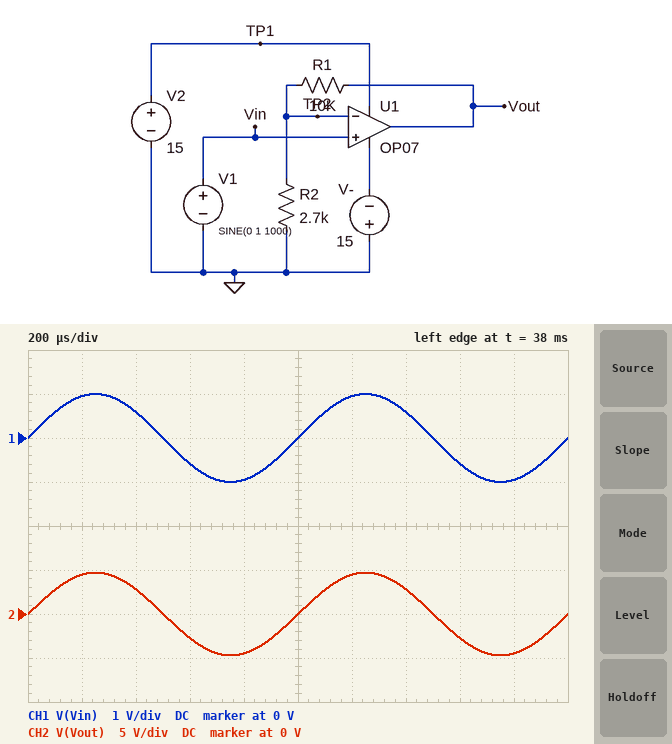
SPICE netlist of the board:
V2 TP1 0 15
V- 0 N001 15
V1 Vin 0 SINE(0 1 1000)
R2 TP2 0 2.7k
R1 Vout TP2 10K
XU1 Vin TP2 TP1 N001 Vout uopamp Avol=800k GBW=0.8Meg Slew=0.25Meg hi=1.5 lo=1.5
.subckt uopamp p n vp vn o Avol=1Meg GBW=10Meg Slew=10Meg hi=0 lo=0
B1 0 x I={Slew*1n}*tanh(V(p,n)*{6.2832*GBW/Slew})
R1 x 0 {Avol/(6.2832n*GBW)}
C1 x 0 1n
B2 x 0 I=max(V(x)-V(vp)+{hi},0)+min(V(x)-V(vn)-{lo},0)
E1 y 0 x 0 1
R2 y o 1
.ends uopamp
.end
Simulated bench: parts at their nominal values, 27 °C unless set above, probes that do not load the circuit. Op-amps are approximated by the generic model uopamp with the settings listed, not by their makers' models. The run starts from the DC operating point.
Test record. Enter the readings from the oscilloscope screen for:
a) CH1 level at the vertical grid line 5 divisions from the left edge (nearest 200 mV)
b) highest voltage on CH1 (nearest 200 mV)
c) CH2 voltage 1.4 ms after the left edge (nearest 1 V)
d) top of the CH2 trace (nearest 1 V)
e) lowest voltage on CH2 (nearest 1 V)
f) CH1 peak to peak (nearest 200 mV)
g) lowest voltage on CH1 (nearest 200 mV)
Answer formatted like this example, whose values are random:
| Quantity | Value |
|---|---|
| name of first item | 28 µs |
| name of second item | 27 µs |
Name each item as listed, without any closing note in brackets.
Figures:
| Quantity | Value |
|---|---|
| CH1 level at the vertical grid line 5 divisions from the left edge | 0 V |
| highest voltage on CH1 | 1.0 V |
| CH2 voltage 1.4 ms after the left edge | 3 V |
| top of the CH2 trace | 5 V |
| lowest voltage on CH2 | -5 V |
| CH1 peak to peak | 2.0 V |
| lowest voltage on CH1 | -1.0 V |
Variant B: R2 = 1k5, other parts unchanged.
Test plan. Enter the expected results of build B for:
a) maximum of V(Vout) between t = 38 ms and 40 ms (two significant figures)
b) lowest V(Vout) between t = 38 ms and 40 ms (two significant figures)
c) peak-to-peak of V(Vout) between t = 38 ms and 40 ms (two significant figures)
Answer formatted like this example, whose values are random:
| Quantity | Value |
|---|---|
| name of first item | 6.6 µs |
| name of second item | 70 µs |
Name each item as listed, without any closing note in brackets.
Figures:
| Quantity | Value |
|---|---|
| maximum of V(Vout) between t = 38 ms and 40 ms | 7.7 V |
| lowest V(Vout) between t = 38 ms and 40 ms | -7.7 V |
| peak-to-peak of V(Vout) between t = 38 ms and 40 ms | 15 V |
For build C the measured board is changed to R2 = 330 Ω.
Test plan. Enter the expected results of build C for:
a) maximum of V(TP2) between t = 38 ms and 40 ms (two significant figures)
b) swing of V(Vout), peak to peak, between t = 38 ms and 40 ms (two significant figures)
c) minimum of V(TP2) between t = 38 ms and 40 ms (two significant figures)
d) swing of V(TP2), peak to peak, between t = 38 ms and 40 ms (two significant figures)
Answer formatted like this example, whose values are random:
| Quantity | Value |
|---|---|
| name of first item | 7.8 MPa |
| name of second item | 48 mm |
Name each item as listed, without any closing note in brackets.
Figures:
| Quantity | Value |
|---|---|
| maximum of V(TP2) between t = 38 ms and 40 ms | 430 mV |
| swing of V(Vout), peak to peak, between t = 38 ms and 40 ms | 27 V |
| minimum of V(TP2) between t = 38 ms and 40 ms | -430 mV |
| swing of V(TP2), peak to peak, between t = 38 ms and 40 ms | 860 mV |
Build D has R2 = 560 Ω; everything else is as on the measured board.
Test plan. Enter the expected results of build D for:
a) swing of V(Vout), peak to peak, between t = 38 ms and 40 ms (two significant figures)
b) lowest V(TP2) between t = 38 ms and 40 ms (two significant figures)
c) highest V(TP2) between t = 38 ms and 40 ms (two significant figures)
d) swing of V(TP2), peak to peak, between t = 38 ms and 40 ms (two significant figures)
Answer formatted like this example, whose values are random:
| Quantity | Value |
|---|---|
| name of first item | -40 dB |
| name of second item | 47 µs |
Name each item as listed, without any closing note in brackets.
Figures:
| Quantity | Value |
|---|---|
| swing of V(Vout), peak to peak, between t = 38 ms and 40 ms | 27 V |
| lowest V(TP2) between t = 38 ms and 40 ms | -720 mV |
| highest V(TP2) between t = 38 ms and 40 ms | 720 mV |
| swing of V(TP2), peak to peak, between t = 38 ms and 40 ms | 1.4 V |
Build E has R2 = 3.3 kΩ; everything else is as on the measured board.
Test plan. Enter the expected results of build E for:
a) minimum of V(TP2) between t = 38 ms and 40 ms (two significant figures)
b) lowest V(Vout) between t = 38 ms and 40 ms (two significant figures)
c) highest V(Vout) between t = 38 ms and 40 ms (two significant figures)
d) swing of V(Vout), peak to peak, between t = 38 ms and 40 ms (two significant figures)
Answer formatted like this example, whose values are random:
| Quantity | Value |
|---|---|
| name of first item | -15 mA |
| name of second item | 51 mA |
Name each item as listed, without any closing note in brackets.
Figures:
| Quantity | Value |
|---|---|
| minimum of V(TP2) between t = 38 ms and 40 ms | -1.0 V |
| lowest V(Vout) between t = 38 ms and 40 ms | -4.0 V |
| highest V(Vout) between t = 38 ms and 40 ms | 4.0 V |
| swing of V(Vout), peak to peak, between t = 38 ms and 40 ms | 8.1 V |
